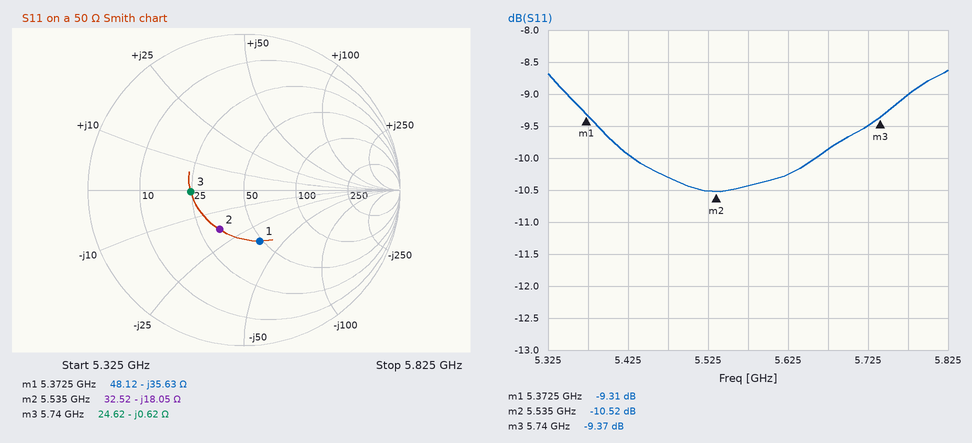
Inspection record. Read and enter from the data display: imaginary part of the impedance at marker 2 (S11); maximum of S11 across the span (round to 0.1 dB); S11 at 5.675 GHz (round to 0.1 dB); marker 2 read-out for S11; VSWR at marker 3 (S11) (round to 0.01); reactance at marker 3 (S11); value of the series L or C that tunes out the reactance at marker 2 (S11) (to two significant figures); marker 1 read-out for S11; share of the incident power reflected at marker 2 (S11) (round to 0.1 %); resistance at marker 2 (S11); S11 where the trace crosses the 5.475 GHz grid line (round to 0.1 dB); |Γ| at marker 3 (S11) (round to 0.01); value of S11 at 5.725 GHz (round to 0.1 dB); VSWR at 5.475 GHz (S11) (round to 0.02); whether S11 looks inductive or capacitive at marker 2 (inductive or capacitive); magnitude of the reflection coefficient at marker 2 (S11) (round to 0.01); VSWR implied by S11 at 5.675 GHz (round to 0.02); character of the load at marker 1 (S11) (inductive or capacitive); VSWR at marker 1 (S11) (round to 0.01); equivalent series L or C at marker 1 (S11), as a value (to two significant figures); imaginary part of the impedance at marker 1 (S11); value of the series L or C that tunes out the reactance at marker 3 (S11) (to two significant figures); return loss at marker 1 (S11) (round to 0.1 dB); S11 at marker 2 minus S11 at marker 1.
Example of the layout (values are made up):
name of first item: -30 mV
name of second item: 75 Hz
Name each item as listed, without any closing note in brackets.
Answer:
imaginary part of the impedance at marker 2: -18.05 Ω
maximum of S11 across the span: -8.6 dB
S11 at 5.675 GHz: -9.9 dB
marker 2 read-out for S11: -10.52 dB
VSWR at marker 3 (S11): 2.03
reactance at marker 3: -0.62 Ω
value of the series L or C that tunes out the reactance at marker 2 (S11): 520 pH
marker 1 read-out for S11: -9.31 dB
share of the incident power reflected at marker 2 (S11): 8.9 %
resistance at marker 2: 32.52 Ω
S11 where the trace crosses the 5.475 GHz grid line: -10.3 dB
|Γ| at marker 3 (S11): 0.34
value of S11 at 5.725 GHz: -9.5 dB
VSWR at 5.475 GHz (S11): 1.88
whether S11 looks inductive or capacitive at marker 2: capacitive
magnitude of the reflection coefficient at marker 2 (S11): 0.30
VSWR implied by S11 at 5.675 GHz: 1.94
character of the load at marker 1 (S11): capacitive
VSWR at marker 1 (S11): 2.04
equivalent series L or C at marker 1 (S11), as a value: 830 fF
imaginary part of the impedance at marker 1: -35.63 Ω
value of the series L or C that tunes out the reactance at marker 3 (S11): 17 pH
return loss at marker 1 (S11): 9.3 dB
S11 at marker 2 minus S11 at marker 1: -1.21 dB
